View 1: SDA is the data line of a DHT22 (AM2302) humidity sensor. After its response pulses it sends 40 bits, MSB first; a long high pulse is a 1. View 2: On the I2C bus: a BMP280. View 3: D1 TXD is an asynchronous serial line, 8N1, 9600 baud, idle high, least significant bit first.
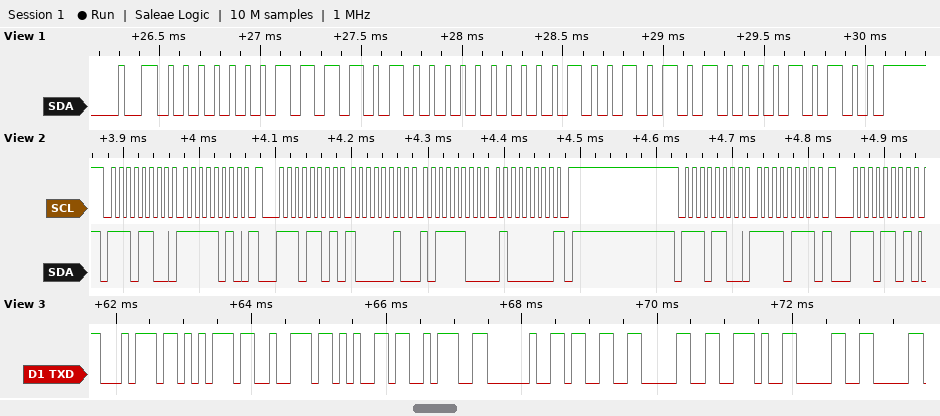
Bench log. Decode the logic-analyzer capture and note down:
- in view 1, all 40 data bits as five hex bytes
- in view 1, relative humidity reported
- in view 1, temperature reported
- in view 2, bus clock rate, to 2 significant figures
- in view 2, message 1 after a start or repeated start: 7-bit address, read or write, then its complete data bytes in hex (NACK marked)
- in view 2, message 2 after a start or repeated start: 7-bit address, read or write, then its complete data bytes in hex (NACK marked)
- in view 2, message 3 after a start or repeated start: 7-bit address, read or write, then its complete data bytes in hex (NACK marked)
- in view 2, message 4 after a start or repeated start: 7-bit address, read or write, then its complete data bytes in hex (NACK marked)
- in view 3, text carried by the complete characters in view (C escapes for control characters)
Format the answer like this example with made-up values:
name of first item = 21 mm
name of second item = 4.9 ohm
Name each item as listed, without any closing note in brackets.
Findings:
in view 1, all 40 data bits as five hex bytes = 01 E8 01 2A 14
in view 1, relative humidity reported = 48.8 %
in view 1, temperature reported = 29.8 °C
in view 2, bus clock rate, to 2 significant figures = 100 kHz
in view 2, message 1 after a start or repeated start: 7-bit address, read or write, then its complete data bytes in hex = 0x76 write: FA
in view 2, message 2 after a start or repeated start: 7-bit address, read or write, then its complete data bytes in hex = 0x76 read: 82 BC 40 NACK
in view 2, message 3 after a start or repeated start: 7-bit address, read or write, then its complete data bytes in hex = 0x76 write: F7
in view 2, message 4 after a start or repeated start: 7-bit address, read or write, then its complete data bytes in hex = 0x76 read
in view 3, text carried by the complete characters in view = "ture: 30.0"
